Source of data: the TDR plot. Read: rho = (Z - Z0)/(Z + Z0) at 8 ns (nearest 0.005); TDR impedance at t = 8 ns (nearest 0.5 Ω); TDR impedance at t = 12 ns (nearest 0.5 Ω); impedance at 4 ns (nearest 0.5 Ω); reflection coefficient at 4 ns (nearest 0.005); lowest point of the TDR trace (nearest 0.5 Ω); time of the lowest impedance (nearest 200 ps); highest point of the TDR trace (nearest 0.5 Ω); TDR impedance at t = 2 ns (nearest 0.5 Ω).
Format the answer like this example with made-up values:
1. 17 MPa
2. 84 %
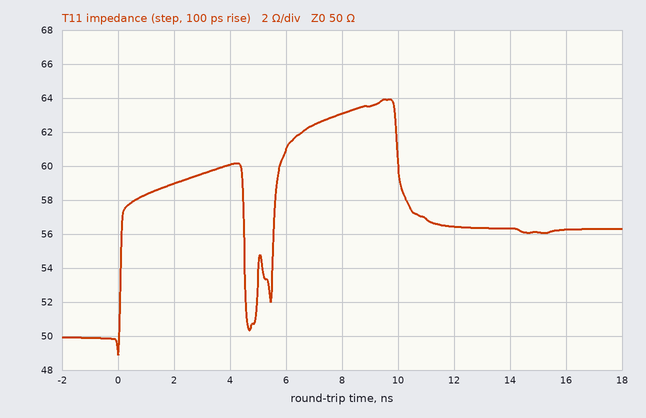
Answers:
1. +0.115
2. 63.0 Ω
3. 56.5 Ω
4. 60.0 Ω
5. +0.090
6. 49.0 Ω
7. 0.0 ns
8. 64.0 Ω
9. 59.0 Ω
